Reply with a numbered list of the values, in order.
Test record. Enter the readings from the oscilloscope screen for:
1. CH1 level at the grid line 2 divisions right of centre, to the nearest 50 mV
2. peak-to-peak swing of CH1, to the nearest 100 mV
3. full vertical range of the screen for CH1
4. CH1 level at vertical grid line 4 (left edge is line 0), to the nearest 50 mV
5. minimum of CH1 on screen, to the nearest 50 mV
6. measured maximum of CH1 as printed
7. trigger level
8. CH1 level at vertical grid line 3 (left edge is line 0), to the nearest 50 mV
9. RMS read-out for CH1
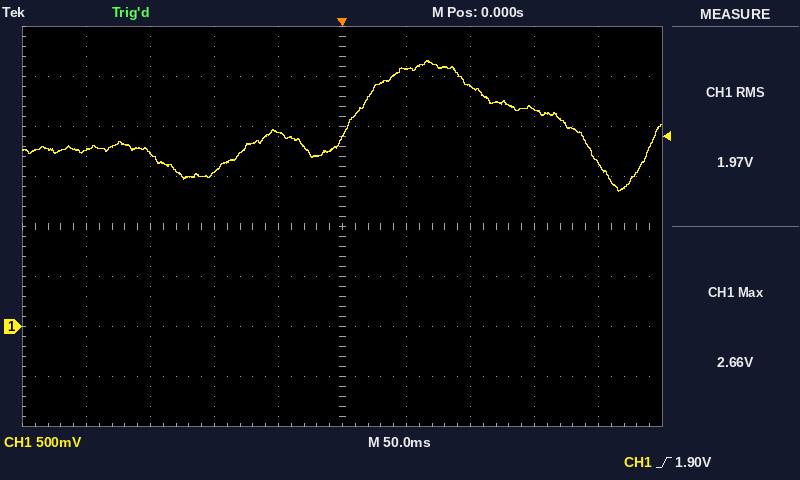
1. 2.40 V
2. 1.30 V
3. 4 V
4. 1.95 V
5. 1.35 V
6. 2.66 V
7. 1.90 V
8. 1.55 V
9. 1.97 V
